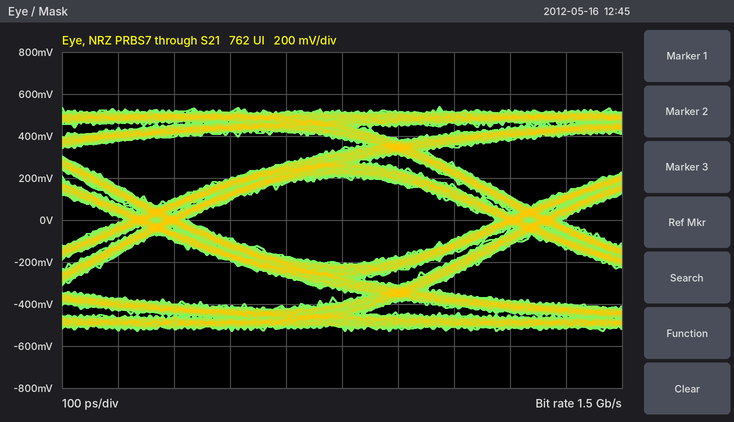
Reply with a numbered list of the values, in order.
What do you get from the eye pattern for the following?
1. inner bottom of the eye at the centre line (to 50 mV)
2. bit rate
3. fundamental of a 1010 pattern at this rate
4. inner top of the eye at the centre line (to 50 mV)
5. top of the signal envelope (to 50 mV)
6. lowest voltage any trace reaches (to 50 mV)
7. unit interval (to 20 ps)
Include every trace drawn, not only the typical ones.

1. -200 mV
2. 1.5 Gb/s
3. 750 MHz
4. 200 mV
5. 550 mV
6. -550 mV
7. 660 ps
